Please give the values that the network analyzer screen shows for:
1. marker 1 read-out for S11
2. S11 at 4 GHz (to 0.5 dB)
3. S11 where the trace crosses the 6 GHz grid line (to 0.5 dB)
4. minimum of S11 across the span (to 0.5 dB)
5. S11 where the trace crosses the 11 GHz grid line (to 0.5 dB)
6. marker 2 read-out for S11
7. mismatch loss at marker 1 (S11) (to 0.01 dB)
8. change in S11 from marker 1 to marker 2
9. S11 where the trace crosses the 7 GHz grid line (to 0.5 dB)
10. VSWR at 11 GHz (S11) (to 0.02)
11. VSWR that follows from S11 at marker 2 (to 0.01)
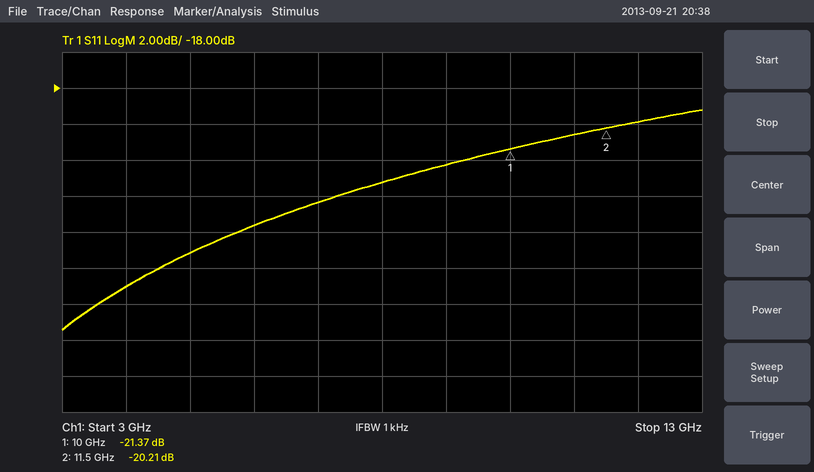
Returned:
-21.37 dB
-29.0 dB
-25.5 dB
-31.5 dB
-20.5 dB
-20.21 dB
0.03 dB
1.16 dB
-24.5 dB
1.20
1.22
